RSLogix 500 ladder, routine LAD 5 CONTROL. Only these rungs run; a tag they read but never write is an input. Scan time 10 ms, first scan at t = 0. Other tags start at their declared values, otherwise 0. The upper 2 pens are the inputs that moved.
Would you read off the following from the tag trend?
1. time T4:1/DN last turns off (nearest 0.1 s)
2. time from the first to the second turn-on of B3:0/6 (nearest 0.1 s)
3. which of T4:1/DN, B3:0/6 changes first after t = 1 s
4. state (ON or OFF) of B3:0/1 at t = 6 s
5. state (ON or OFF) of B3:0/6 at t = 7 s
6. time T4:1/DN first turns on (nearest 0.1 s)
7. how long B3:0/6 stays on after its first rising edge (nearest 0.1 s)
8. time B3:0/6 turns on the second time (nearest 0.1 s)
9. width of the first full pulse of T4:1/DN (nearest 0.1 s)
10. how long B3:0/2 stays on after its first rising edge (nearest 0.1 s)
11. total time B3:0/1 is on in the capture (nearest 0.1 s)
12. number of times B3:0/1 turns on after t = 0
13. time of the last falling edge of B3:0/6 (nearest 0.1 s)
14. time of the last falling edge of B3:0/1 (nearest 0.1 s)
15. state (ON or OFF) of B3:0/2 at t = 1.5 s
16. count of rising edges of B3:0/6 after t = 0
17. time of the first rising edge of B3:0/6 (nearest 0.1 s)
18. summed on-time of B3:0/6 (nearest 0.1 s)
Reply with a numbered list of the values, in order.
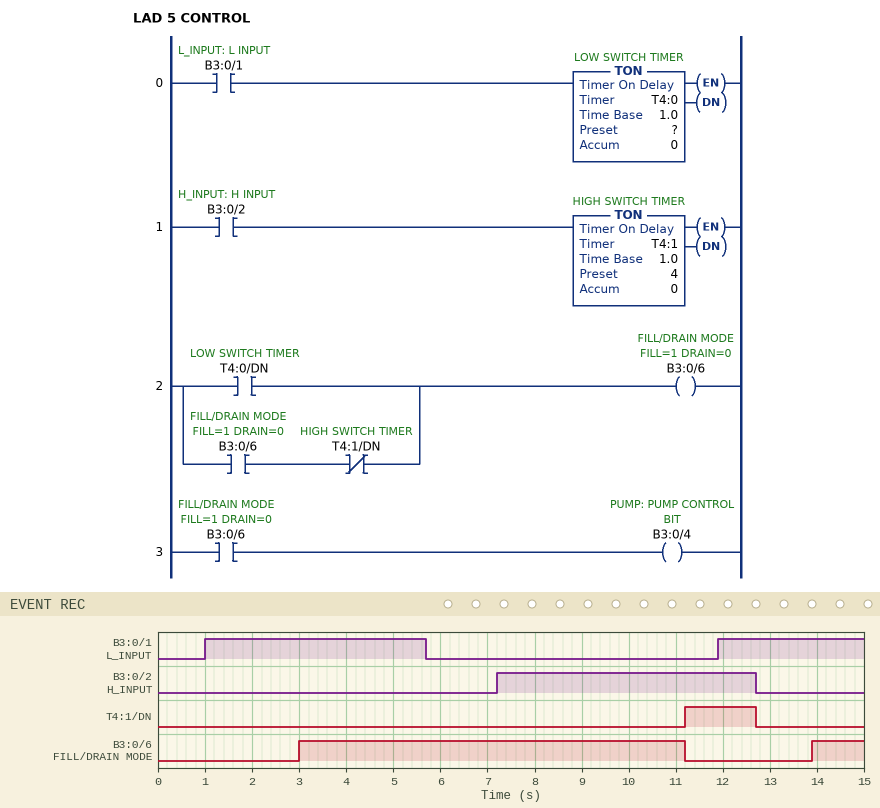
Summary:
1. 12.7 s
2. 10.9 s
3. B3:0/6
4. OFF
5. ON
6. 11.2 s
7. 8.2 s
8. 13.9 s
9. 1.5 s
10. 5.5 s
11. 7.8 s
12. 2
13. 11.2 s
14. 5.7 s
15. OFF
16. 2
17. 3.0 s
18. 9.3 s
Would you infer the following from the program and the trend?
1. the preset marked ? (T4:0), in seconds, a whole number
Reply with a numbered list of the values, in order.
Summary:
1. 2 s
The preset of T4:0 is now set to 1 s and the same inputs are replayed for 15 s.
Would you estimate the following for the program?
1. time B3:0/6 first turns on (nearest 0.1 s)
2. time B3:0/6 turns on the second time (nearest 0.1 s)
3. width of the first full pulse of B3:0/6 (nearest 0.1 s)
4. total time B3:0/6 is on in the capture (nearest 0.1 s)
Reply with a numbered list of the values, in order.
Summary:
1. 2.0 s
2. 12.9 s
3. 9.2 s
4. 11.3 s
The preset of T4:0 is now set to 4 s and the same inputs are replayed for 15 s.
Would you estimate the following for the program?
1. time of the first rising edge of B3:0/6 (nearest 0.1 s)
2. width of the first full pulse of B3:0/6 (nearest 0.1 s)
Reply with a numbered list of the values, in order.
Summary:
1. 5.0 s
2. 6.2 s
